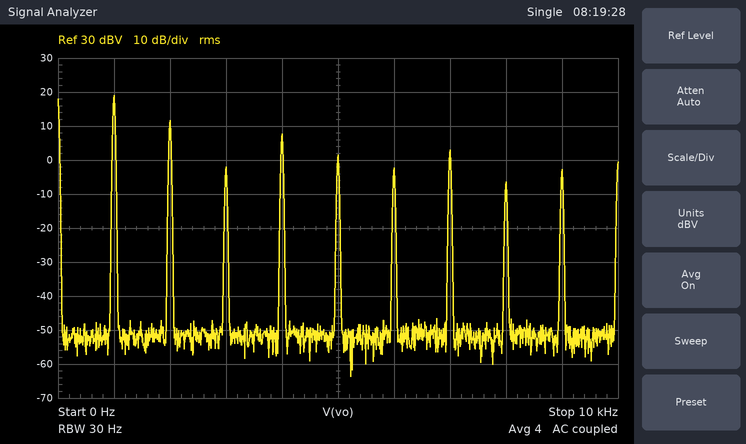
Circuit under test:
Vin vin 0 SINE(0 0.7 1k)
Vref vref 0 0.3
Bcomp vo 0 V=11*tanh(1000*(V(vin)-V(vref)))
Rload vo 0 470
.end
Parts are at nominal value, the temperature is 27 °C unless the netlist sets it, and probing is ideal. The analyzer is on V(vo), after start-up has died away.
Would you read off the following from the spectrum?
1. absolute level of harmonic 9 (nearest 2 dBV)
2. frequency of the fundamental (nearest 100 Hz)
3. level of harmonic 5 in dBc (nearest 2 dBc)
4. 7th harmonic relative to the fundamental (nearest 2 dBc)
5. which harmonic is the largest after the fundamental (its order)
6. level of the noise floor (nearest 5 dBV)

-2 dBV
1.0 kHz
-18 dBc
-16 dBc
2
-50 dBV
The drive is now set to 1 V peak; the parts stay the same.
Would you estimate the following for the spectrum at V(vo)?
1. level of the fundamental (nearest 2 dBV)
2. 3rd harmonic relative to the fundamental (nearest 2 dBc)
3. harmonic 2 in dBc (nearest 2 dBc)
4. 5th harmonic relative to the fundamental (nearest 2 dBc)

20 dBV
-14 dBc
-10 dBc
-40 dBc
